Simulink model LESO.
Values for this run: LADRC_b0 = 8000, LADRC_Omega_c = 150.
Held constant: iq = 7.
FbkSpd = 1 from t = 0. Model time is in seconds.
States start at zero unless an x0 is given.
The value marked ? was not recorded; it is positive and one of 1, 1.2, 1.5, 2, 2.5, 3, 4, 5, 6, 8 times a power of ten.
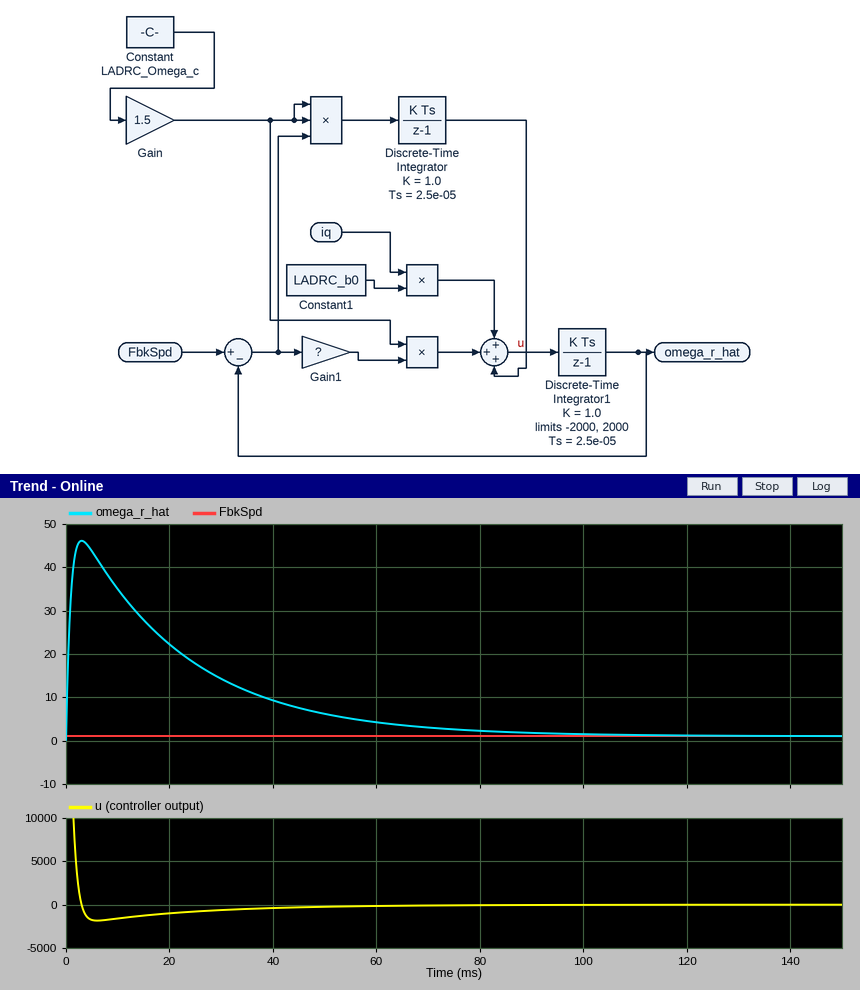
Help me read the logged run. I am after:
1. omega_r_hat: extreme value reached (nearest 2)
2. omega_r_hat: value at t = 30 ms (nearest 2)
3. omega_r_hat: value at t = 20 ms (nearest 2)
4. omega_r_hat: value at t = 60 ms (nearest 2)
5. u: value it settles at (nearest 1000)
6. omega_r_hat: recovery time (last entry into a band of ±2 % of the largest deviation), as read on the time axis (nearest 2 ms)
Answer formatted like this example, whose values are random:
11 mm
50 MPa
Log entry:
46
14
22
4
0
86 ms
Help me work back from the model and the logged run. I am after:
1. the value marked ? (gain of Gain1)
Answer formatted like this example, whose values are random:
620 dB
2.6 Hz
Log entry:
5
